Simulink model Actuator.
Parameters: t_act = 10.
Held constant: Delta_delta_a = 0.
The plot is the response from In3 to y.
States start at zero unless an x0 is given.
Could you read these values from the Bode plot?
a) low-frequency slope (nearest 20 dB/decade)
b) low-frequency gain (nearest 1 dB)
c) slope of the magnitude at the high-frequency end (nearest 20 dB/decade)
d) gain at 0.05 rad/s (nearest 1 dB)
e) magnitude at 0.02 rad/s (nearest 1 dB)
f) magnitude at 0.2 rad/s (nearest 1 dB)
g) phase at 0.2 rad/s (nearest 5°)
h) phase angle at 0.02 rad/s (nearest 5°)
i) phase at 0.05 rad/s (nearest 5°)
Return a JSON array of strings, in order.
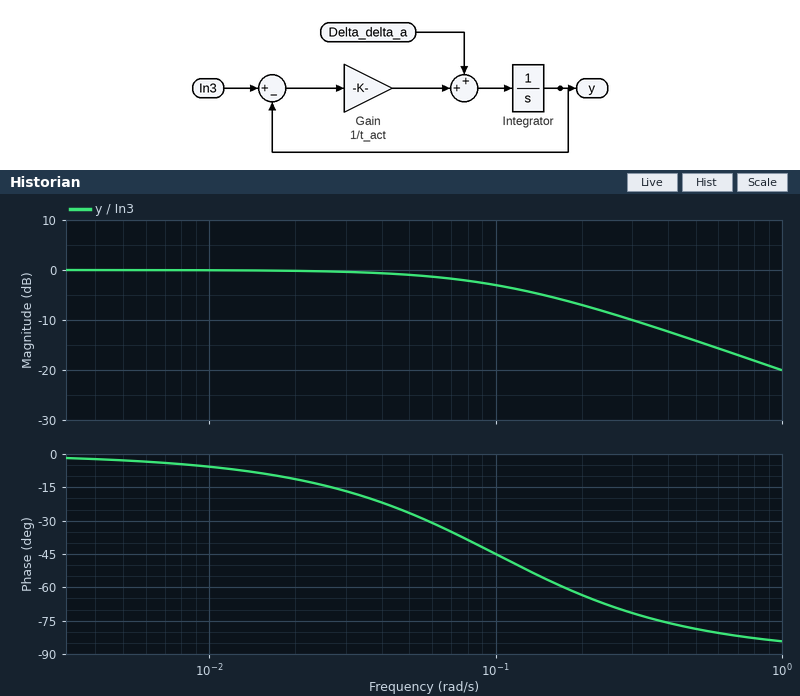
["0 dB/decade", "0 dB", "-20 dB/decade", "-1 dB", "0 dB", "-7 dB", "-65°", "-10°", "-25°"]
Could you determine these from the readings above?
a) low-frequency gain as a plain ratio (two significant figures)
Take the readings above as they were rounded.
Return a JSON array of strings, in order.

["1.0"]
